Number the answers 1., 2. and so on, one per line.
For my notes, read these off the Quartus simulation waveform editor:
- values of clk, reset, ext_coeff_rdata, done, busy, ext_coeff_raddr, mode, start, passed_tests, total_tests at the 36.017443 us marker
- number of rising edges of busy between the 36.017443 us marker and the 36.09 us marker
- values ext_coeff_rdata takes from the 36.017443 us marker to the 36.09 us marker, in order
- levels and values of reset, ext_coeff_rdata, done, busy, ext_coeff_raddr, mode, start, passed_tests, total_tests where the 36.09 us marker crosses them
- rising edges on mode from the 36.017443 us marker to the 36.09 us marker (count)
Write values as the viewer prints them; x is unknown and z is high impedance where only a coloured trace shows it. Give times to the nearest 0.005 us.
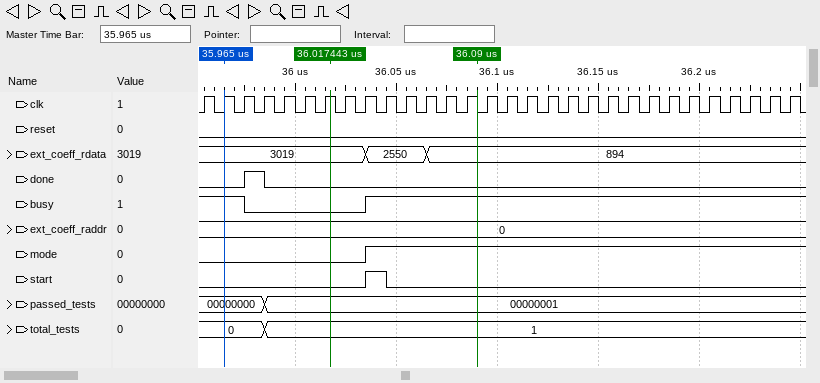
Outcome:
1. clk=1, reset=0, ext_coeff_rdata=3019, done=0, busy=0, ext_coeff_raddr=0, mode=0, start=0, passed_tests=00000001, total_tests=1
2. 1
3. 3019, 2550, 894
4. reset=0, ext_coeff_rdata=894, done=0, busy=1, ext_coeff_raddr=0, mode=1, start=0, passed_tests=00000001, total_tests=1
5. 1
